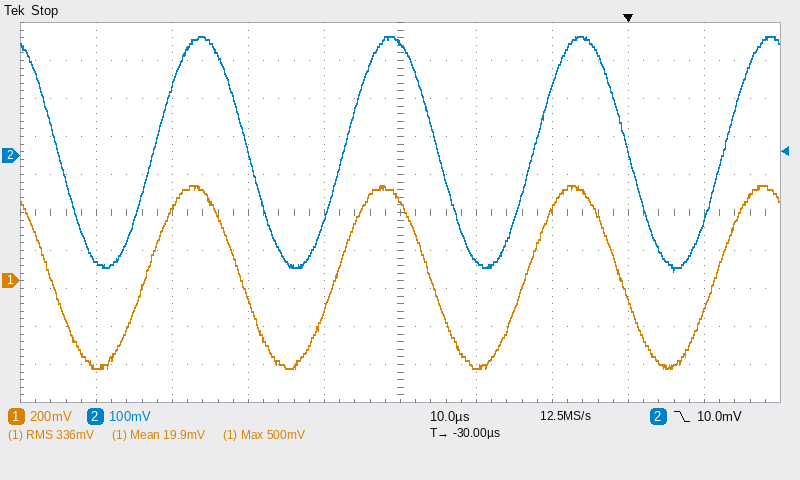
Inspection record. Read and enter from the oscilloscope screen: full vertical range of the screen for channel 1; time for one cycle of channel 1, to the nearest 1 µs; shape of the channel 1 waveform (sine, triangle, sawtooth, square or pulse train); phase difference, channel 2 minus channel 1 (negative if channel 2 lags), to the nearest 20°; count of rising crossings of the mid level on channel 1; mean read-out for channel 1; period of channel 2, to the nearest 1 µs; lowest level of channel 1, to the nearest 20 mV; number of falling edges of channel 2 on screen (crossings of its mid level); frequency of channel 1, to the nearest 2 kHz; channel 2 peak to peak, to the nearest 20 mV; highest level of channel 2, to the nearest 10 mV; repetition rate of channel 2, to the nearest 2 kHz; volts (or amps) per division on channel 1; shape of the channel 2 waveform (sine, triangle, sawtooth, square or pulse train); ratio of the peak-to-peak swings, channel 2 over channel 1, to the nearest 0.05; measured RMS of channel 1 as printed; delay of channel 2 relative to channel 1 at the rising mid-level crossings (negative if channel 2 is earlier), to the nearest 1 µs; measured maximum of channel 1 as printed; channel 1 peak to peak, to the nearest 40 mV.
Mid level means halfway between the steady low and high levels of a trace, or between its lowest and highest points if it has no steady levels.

2 V
25 µs
sine
-20°
4
19.9 mV
25 µs
-460 mV
4
40 kHz
620 mV
310 mV
40 kHz
200 mV
sine
0.65
336 mV
+1 µs
500 mV
960 mV
